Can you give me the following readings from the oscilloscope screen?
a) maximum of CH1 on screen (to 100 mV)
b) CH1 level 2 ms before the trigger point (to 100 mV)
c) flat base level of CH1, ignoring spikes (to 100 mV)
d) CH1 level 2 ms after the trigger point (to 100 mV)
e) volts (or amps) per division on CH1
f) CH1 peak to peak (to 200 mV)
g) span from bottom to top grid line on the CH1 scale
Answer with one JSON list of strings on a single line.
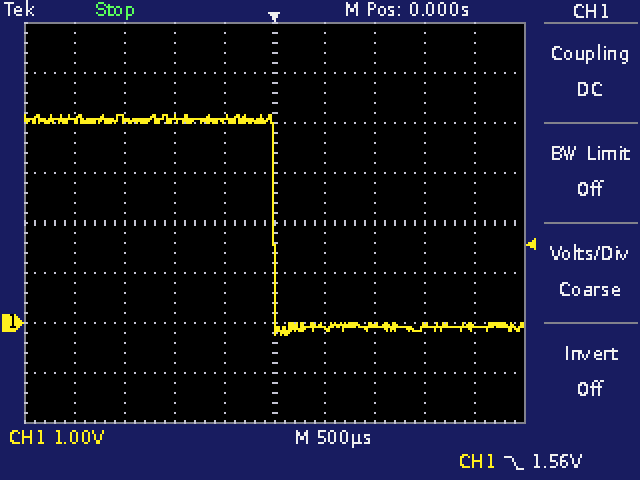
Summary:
["4.2 V", "4.1 V", "-100 mV", "-100 mV", "1 V", "4.4 V", "8 V"]
